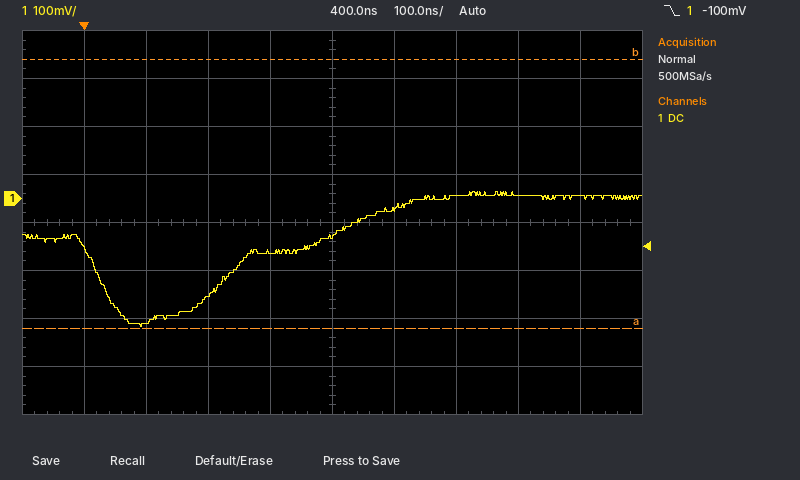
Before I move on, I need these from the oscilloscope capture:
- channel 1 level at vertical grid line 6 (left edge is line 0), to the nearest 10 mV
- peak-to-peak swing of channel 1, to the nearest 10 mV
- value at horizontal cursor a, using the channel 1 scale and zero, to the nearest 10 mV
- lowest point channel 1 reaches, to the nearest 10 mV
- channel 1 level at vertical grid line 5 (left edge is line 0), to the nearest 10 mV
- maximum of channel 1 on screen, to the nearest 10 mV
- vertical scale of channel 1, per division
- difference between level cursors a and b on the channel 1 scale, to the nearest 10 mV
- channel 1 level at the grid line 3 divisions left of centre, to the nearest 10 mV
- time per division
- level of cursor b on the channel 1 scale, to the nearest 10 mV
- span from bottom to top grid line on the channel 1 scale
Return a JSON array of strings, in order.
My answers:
["-20 mV", "280 mV", "-270 mV", "-270 mV", "-80 mV", "10 mV", "100 mV", "560 mV", "-260 mV", "100 ns", "290 mV", "800 mV"]
